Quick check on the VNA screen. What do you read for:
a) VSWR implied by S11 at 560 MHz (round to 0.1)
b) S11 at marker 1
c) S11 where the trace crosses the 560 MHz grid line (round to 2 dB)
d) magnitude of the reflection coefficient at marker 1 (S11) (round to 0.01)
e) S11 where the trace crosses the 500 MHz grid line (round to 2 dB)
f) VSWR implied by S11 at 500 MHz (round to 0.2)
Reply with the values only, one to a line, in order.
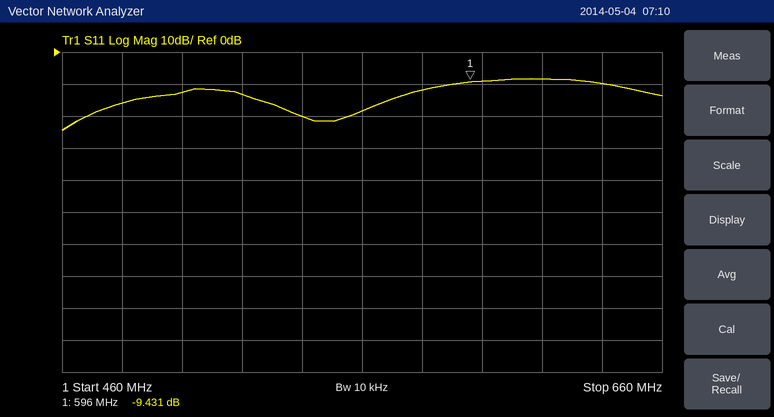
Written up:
1.3
-9.431 dB
-18 dB
0.34
-12 dB
1.6
